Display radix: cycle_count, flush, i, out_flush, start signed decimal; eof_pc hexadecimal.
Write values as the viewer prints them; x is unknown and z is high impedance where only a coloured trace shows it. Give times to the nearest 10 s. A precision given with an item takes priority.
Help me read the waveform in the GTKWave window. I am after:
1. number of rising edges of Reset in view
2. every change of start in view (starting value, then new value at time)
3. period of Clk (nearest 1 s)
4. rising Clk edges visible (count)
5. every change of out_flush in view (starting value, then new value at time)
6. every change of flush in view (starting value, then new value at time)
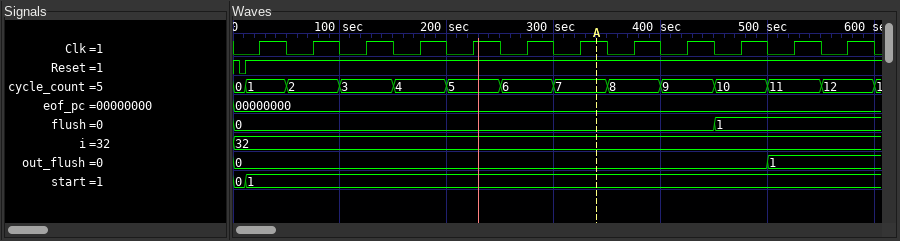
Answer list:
1
0, 1 at 10 s
50 s
12
0, 1 at 500 s
0, 1 at 450 s
